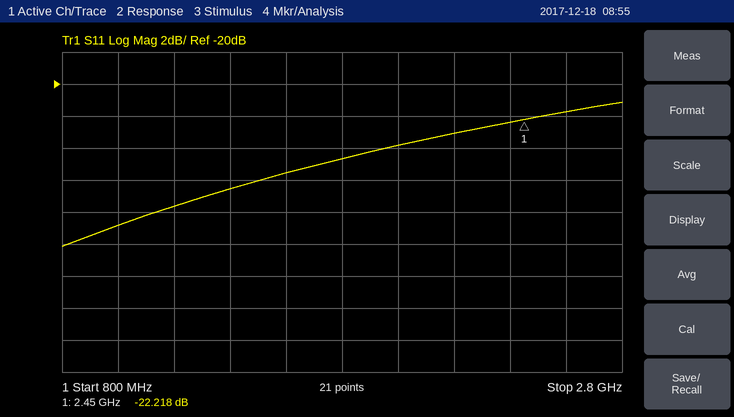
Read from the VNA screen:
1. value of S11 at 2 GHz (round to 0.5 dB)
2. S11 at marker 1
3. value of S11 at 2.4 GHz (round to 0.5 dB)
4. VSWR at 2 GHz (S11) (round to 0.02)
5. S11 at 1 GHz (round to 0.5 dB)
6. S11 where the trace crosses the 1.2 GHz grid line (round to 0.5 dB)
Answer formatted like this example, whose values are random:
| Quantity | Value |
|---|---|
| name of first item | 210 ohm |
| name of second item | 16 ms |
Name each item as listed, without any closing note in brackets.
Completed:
| Quantity | Value |
|---|---|
| value of S11 at 2 GHz | -24.0 dB |
| S11 at marker 1 | -22.218 dB |
| value of S11 at 2.4 GHz | -22.5 dB |
| VSWR at 2 GHz (S11) | 1.14 |
| S11 at 1 GHz | -29.0 dB |
| S11 where the trace crosses the 1.2 GHz grid line | -27.5 dB |
